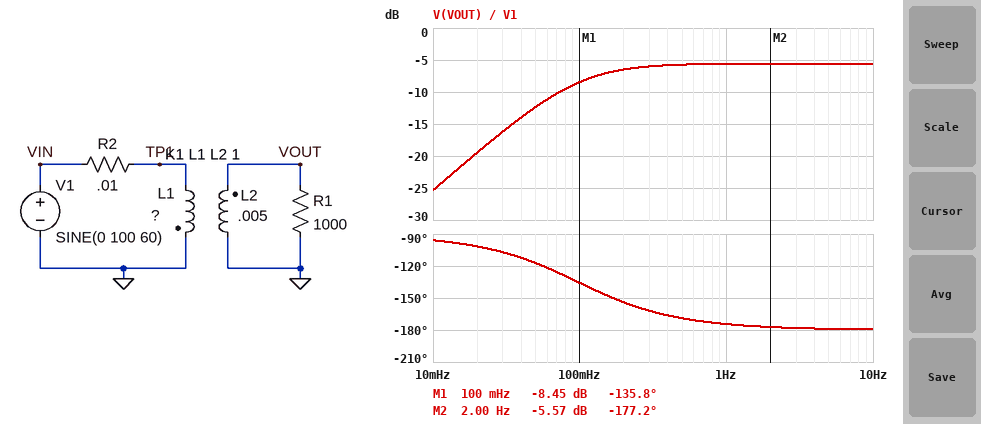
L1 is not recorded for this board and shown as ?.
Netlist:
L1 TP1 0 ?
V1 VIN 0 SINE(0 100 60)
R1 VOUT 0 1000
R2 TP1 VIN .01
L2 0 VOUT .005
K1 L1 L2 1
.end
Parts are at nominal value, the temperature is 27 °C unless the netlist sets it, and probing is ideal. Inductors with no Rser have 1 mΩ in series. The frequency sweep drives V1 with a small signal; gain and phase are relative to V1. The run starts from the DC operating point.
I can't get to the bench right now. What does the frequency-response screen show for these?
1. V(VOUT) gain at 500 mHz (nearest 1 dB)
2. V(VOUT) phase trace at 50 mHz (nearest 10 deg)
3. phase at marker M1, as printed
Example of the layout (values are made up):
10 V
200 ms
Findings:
-6 dB
-120 deg
-135.8 deg
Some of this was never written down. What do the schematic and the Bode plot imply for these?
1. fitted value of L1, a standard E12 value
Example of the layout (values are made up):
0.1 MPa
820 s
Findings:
18 mH
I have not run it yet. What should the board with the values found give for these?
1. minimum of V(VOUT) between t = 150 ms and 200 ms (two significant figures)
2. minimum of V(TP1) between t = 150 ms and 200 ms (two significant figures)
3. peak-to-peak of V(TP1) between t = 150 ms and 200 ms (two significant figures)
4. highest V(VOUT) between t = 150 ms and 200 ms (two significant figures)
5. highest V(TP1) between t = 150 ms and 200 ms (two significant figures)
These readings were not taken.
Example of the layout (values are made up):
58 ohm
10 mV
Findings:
-53 V
-100 V
200 V
53 V
100 V
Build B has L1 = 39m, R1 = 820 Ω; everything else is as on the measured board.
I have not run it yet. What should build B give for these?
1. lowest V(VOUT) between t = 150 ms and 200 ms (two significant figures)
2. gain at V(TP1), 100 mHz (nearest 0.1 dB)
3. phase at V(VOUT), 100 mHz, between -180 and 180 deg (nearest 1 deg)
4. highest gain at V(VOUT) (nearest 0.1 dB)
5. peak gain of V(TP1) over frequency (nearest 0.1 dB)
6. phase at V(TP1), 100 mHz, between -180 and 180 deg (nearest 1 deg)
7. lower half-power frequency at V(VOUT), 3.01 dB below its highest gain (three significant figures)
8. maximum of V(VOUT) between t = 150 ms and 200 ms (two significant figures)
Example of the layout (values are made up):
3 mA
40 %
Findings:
-36 V
-0.8 dB
-156 deg
-8.9 dB
0 dB
22 deg
44.9 mHz
36 V
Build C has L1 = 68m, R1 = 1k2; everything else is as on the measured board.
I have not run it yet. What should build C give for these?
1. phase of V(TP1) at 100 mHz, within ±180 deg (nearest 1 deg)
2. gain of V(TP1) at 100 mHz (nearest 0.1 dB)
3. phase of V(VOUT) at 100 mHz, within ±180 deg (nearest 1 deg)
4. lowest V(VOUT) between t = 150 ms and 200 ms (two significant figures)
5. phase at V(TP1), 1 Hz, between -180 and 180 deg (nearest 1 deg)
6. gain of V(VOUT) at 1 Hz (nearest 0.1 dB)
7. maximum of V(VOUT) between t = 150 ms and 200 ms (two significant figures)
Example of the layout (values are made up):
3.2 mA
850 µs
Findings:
13 deg
-0.3 dB
-166 deg
-27 V
1 deg
-11.3 dB
27 V
